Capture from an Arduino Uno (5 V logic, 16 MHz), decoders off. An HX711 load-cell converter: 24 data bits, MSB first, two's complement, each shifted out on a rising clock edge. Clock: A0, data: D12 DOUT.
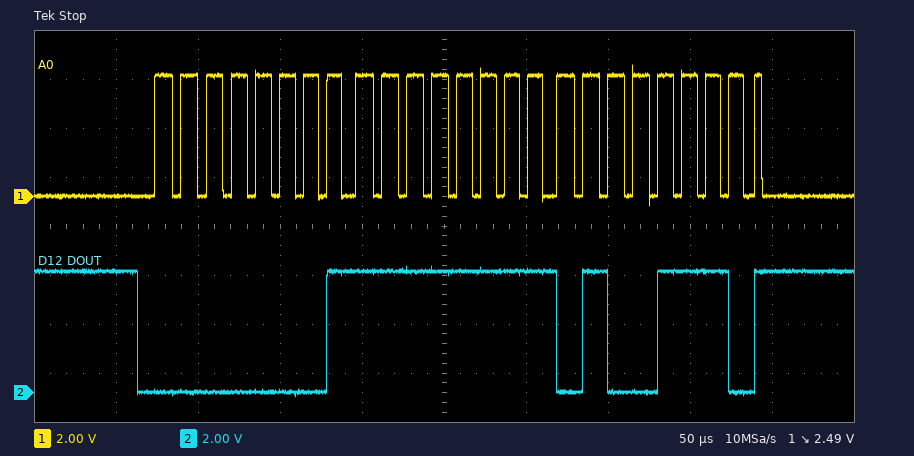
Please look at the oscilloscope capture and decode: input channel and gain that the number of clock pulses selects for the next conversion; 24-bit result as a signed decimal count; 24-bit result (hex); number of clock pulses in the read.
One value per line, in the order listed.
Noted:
channel A, gain 128
130894
0x01FF4E
25
